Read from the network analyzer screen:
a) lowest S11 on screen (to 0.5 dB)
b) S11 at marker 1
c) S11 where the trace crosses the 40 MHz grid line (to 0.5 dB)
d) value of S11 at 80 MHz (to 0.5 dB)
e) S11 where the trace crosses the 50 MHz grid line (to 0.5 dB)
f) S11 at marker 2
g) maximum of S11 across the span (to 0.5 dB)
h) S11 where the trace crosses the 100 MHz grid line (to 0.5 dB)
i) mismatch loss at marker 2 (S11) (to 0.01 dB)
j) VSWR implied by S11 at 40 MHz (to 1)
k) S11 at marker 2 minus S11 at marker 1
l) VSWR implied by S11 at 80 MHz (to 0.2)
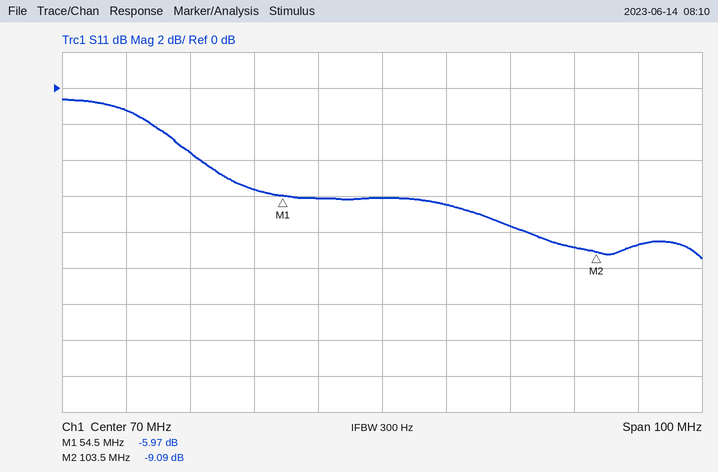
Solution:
-9.5 dB
-5.97 dB
-3.5 dB
-6.5 dB
-5.5 dB
-9.09 dB
-0.5 dB
-9.0 dB
0.57 dB
5
-3.12 dB
2.8
